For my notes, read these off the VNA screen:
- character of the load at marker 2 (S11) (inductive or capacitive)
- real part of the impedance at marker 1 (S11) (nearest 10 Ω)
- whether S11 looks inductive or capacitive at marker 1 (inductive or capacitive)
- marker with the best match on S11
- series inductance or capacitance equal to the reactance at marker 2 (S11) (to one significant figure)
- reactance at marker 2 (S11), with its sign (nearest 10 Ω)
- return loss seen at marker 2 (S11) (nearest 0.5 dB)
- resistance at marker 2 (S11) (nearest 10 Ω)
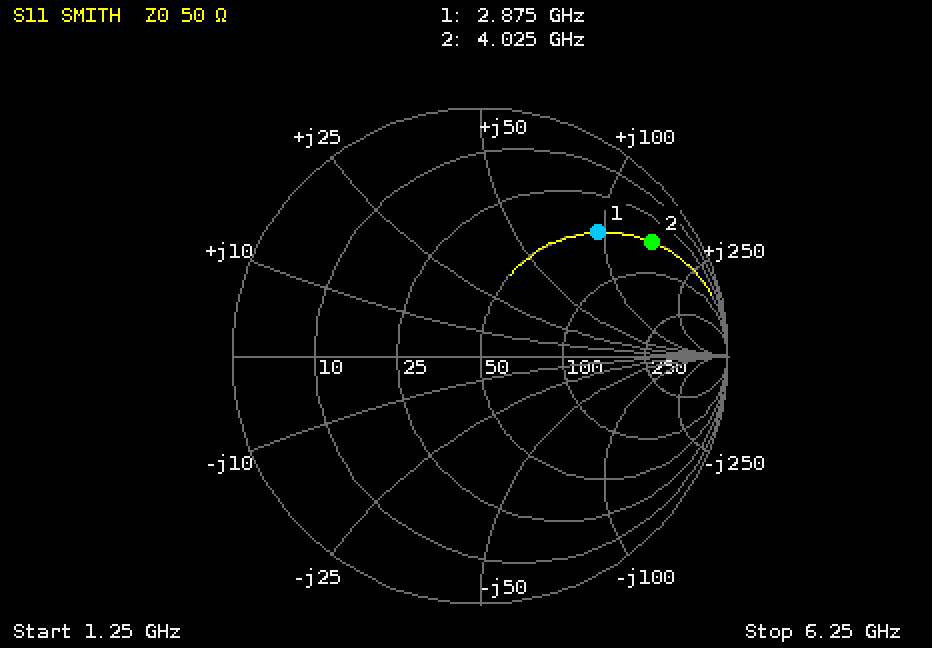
inductive
50 Ω
inductive
marker 1
6 nH
+150 Ω
1.5 dB
50 Ω
